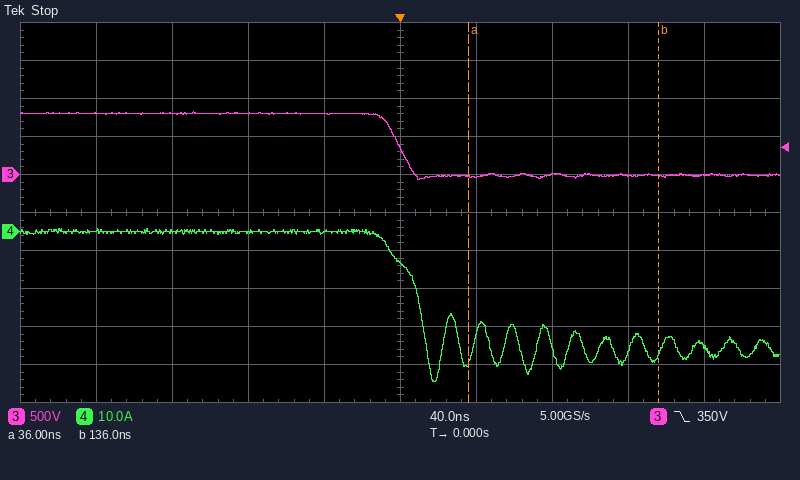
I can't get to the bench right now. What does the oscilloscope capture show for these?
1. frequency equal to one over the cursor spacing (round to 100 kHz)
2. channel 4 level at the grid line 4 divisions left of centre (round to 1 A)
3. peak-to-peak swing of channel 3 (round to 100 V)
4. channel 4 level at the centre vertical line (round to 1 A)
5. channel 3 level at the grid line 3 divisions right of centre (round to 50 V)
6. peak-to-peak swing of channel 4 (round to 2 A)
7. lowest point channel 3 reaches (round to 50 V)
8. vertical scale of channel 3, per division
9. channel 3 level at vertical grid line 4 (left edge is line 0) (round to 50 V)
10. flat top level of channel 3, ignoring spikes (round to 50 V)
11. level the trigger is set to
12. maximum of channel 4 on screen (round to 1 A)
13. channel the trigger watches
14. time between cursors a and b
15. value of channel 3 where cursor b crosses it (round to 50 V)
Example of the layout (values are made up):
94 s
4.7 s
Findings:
10.0 MHz
0 A
900 V
-8 A
0 V
40 A
-50 V
500 V
800 V
800 V
350 V
1 A
channel 3
100 ns
0 V
